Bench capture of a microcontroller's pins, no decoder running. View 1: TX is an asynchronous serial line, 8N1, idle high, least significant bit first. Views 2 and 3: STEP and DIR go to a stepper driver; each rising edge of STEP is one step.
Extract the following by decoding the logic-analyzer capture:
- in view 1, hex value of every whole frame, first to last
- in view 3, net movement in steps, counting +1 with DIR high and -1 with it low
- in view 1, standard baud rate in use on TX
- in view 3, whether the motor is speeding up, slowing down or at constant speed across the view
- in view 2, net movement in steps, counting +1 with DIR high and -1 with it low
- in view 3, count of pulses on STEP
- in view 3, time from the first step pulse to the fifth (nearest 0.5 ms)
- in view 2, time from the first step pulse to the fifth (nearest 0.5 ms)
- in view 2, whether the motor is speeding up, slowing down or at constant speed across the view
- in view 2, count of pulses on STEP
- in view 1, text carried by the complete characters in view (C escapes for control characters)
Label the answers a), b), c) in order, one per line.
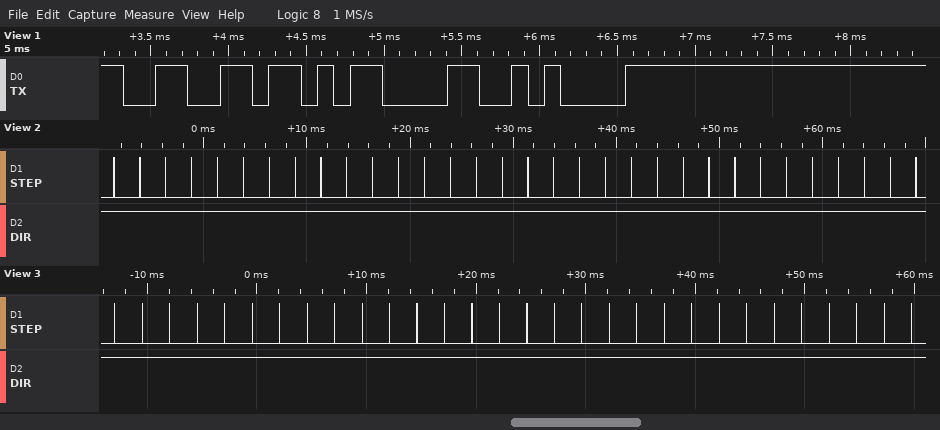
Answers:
a) 66 0D 0A
b) +30
c) 9600 baud
d) constant speed
e) +32
f) 30
g) 10.0 ms
h) 10.0 ms
i) constant speed
j) 32
k) "f\r\n"
